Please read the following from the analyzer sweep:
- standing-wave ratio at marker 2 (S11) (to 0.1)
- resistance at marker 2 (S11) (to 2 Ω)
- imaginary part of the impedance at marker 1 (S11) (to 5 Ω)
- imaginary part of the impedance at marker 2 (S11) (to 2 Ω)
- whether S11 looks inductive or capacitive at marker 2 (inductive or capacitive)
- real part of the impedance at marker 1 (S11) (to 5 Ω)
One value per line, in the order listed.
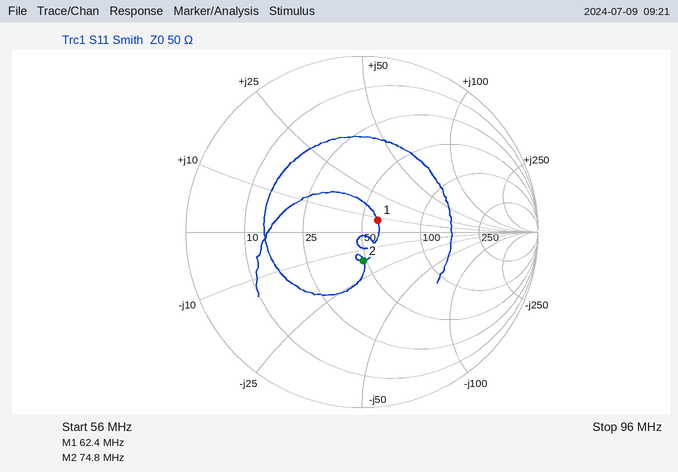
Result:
1.4
48 Ω
+10 Ω
-16 Ω
capacitive
60 Ω
